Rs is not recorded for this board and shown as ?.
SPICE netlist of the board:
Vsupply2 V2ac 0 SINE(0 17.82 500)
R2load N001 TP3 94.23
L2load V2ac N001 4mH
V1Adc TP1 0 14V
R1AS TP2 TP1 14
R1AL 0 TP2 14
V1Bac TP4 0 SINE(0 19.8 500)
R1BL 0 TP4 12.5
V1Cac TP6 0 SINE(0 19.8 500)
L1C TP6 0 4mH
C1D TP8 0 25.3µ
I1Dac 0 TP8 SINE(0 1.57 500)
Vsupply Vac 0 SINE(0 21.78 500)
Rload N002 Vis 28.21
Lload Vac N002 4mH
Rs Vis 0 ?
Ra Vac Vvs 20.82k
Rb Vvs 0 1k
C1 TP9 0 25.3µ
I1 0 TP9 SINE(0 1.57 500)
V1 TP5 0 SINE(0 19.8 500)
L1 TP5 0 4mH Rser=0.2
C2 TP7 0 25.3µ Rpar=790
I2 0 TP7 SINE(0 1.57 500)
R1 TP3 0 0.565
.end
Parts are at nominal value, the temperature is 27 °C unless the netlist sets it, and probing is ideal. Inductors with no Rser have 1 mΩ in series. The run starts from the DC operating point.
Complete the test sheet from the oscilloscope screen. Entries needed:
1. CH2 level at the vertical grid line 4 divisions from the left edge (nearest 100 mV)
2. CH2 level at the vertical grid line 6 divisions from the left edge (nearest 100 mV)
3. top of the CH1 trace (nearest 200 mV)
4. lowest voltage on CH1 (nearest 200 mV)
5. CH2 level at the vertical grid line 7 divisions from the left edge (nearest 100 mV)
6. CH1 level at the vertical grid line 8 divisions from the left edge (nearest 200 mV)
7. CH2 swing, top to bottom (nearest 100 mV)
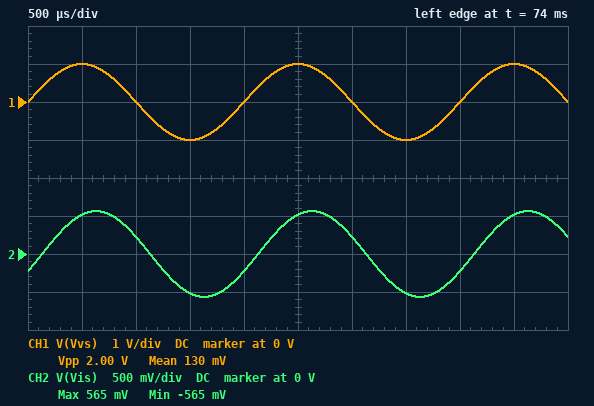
-200 mV
200 mV
1.0 V
-1.0 V
-500 mV
0 V
1.1 V
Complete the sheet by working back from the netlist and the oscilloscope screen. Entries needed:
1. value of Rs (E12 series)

0.82 Ω
